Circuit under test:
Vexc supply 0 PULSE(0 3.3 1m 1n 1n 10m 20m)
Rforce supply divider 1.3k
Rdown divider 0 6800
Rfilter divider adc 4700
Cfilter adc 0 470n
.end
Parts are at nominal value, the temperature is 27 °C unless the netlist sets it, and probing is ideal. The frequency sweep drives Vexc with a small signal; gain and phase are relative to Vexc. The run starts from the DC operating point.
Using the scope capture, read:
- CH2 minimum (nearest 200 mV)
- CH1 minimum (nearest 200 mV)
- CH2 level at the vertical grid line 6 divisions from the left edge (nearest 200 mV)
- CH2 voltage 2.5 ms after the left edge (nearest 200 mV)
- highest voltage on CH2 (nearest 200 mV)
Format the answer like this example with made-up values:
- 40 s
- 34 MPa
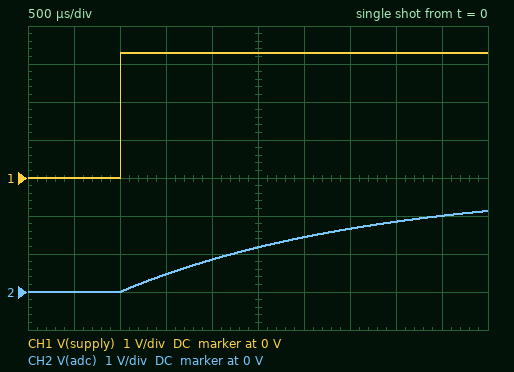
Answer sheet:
- 0 V
- 0 V
- 1.4 V
- 1.2 V
- 2.2 V
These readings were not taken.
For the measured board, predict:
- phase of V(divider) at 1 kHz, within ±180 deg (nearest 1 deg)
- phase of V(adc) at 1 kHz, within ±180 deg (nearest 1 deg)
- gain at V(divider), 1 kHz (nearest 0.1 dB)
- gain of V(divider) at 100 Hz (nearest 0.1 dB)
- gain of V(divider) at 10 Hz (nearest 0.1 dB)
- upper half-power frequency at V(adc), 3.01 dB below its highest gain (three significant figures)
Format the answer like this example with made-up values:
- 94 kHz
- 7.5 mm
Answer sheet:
- -1 deg
- -87 deg
- -3.3 dB
- -2.8 dB
- -1.6 dB
- 58.5 Hz
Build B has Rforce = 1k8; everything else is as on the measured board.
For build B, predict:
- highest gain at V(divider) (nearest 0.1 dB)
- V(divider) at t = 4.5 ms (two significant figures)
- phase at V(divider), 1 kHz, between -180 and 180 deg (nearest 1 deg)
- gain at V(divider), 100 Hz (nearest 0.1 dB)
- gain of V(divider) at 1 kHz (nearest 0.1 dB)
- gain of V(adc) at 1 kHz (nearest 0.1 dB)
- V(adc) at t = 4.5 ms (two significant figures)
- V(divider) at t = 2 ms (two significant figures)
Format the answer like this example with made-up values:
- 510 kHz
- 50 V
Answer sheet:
- -2.0 dB
- 2.4 V
- -1 deg
- -3.7 dB
- -4.3 dB
- -27.2 dB
- 1.8 V
- 2.2 V
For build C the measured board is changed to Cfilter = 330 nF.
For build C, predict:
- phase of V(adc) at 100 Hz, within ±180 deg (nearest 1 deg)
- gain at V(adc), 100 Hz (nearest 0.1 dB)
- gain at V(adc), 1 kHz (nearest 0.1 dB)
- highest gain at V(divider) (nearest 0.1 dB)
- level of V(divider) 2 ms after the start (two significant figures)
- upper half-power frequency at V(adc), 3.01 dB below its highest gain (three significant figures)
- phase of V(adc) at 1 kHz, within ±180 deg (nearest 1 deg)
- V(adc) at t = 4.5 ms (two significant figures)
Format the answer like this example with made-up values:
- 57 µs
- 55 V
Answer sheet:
- -50 deg
- -5.4 dB
- -23.1 dB
- -1.5 dB
- 2.5 V
- 83.3 Hz
- -85 deg
- 2.3 V
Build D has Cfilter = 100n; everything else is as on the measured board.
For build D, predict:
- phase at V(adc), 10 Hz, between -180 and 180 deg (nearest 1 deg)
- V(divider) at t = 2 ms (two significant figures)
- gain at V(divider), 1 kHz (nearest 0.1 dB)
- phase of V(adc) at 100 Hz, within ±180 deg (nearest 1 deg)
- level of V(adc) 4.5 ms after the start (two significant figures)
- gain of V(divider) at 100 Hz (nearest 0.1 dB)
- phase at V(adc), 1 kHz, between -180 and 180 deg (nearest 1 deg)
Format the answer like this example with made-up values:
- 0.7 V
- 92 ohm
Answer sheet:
- -2 deg
- 2.7 V
- -3.2 dB
- -20 deg
- 2.8 V
- -1.7 dB
- -75 deg
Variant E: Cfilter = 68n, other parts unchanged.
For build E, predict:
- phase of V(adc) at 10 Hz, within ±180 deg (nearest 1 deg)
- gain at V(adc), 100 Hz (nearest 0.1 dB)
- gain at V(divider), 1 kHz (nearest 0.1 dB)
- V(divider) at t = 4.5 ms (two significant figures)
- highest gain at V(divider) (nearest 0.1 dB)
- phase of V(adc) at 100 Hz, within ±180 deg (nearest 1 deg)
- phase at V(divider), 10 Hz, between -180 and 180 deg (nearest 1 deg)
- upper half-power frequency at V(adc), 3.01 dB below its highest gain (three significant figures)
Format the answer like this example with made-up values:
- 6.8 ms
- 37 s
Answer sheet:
- -1 deg
- -1.8 dB
- -3.0 dB
- 2.8 V
- -1.5 dB
- -14 deg
- 0 deg
- 404 Hz
